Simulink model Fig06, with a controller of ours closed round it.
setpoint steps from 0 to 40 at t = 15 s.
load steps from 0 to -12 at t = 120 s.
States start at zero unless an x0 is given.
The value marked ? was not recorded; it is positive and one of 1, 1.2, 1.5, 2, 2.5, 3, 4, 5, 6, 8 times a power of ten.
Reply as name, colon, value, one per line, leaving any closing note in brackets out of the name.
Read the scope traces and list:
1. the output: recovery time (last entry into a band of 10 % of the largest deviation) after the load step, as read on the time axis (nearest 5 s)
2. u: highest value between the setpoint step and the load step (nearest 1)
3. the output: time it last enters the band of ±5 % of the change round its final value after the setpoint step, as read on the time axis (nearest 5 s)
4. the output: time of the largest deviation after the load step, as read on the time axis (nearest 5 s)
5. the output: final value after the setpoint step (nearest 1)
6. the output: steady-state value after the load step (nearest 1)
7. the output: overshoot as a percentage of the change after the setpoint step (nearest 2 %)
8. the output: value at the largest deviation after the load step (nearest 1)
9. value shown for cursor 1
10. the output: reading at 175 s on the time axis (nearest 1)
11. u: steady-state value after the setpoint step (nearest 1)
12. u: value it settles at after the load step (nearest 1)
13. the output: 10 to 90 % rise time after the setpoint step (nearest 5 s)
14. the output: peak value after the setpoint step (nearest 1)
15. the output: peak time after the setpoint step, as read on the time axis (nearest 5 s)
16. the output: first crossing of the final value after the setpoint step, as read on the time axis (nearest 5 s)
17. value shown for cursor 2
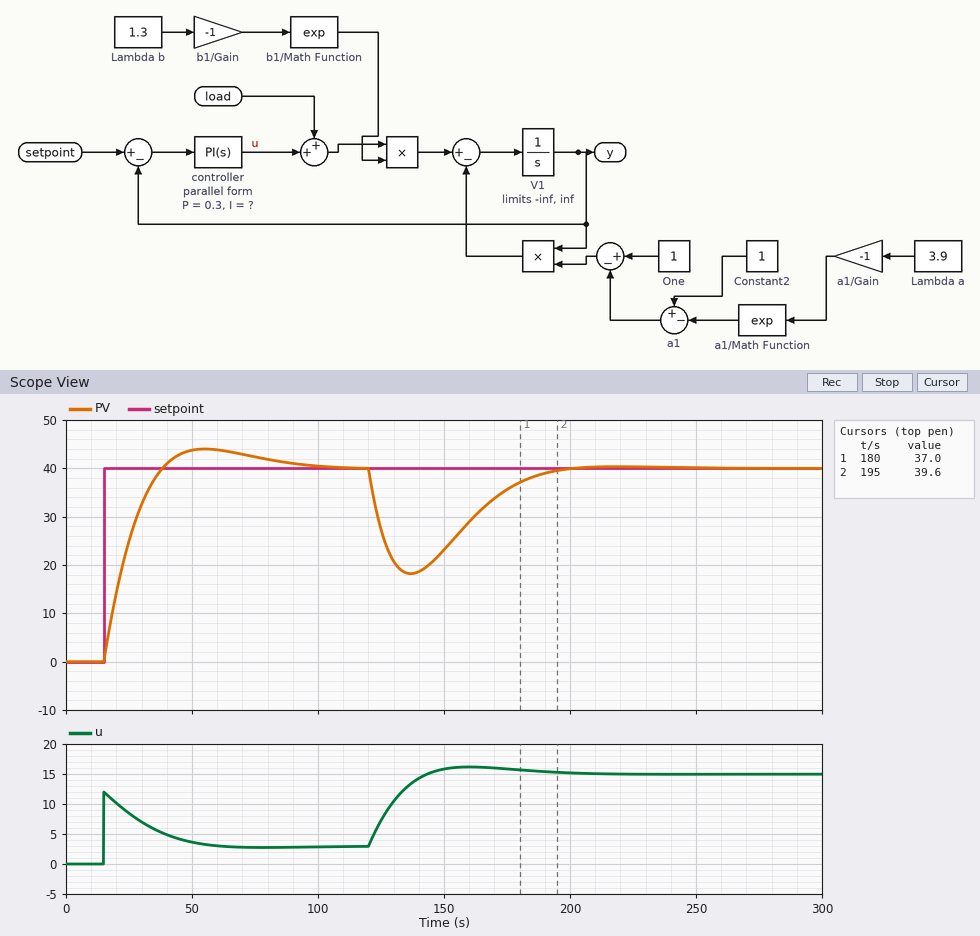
the output: recovery time (last entry into a band of 10 % of the largest deviation) after the load step, as read on the time axis: 185 s
u: highest value between the setpoint step and the load step: 12
the output: time it last enters the band of ±5 % of the change round its final value after the setpoint step, as read on the time axis: 80 s
the output: time of the largest deviation after the load step, as read on the time axis: 135 s
the output: final value after the setpoint step: 40
the output: steady-state value after the load step: 40
the output: overshoot as a percentage of the change after the setpoint step: 10 %
the output: value at the largest deviation after the load step: 18
value shown for cursor 1: 37.0
the output: reading at 175 s on the time axis: 36
u: steady-state value after the setpoint step: 3
u: value it settles at after the load step: 15
the output: 10 to 90 % rise time after the setpoint step: 15 s
the output: peak value after the setpoint step: 44
the output: peak time after the setpoint step, as read on the time axis: 55 s
the output: first crossing of the final value after the setpoint step, as read on the time axis: 40 s
value shown for cursor 2: 39.6
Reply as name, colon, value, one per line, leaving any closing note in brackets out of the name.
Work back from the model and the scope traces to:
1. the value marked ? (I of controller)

the value marked ?: 0.015
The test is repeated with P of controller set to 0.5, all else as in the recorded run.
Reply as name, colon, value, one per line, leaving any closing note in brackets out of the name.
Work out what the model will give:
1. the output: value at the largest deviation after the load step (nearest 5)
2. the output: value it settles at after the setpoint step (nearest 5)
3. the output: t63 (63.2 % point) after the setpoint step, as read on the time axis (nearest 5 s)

the output: value at the largest deviation after the load step: 25
the output: value it settles at after the setpoint step: 40
the output: t63 (63.2 % point) after the setpoint step, as read on the time axis: 20 s
